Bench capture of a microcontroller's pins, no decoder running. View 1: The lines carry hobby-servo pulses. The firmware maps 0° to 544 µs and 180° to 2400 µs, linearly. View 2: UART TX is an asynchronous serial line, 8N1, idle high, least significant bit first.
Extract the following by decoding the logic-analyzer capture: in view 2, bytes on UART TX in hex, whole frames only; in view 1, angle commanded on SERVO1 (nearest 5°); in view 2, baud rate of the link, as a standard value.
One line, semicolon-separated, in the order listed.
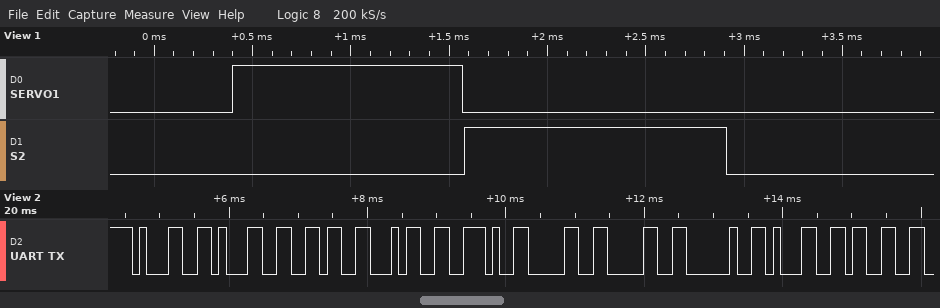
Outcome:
31 31 36 34 2E 30 30 20 31 33; 60°; 9600 baud
